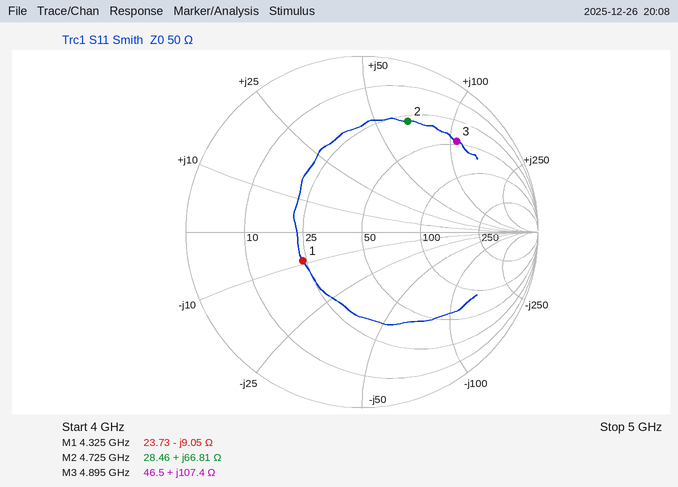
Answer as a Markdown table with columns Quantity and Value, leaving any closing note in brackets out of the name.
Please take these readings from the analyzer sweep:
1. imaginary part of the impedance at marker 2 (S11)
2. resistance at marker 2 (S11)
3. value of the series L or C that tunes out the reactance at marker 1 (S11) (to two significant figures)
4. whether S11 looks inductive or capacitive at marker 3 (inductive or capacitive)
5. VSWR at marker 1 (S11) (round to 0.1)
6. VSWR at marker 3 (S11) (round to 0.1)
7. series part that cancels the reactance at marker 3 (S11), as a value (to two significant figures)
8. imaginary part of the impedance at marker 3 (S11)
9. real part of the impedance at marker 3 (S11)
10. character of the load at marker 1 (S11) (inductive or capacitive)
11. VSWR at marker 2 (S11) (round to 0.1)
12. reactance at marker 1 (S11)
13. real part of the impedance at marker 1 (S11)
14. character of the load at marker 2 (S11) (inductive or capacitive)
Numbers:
| Quantity | Value |
|---|---|
| imaginary part of the impedance at marker 2 | +66.81 Ω |
| resistance at marker 2 | 28.46 Ω |
| value of the series L or C that tunes out the reactance at marker 1 (S11) | 330 pH |
| whether S11 looks inductive or capacitive at marker 3 | inductive |
| VSWR at marker 1 (S11) | 2.2 |
| VSWR at marker 3 (S11) | 6.8 |
| series part that cancels the reactance at marker 3 (S11), as a value | 300 fF |
| imaginary part of the impedance at marker 3 | +107.4 Ω |
| real part of the impedance at marker 3 | 46.5 Ω |
| character of the load at marker 1 (S11) | capacitive |
| VSWR at marker 2 (S11) | 5.3 |
| reactance at marker 1 | -9.05 Ω |
| real part of the impedance at marker 1 | 23.73 Ω |
| character of the load at marker 2 (S11) | inductive |
